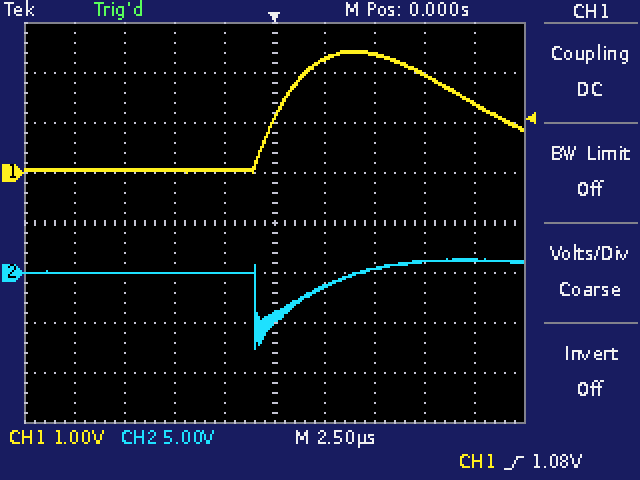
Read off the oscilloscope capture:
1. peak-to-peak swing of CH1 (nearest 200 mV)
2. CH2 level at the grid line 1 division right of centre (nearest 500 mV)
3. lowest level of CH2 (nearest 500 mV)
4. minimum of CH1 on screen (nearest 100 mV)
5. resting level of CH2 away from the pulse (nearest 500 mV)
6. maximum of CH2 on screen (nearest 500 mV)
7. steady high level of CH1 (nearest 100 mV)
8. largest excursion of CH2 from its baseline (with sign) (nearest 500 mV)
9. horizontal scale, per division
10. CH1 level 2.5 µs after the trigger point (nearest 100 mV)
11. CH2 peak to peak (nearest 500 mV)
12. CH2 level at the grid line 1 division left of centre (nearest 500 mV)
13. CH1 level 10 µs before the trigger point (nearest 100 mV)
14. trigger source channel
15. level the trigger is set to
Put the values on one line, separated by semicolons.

2.4 V; -1.5 V; -7.5 V; 0.0 V; 0.0 V; 1.5 V; 2.4 V; -7.5 V; 2.5 µs; 2.3 V; 9.0 V; 0.0 V; 100 mV; CH1; 1.08 V
